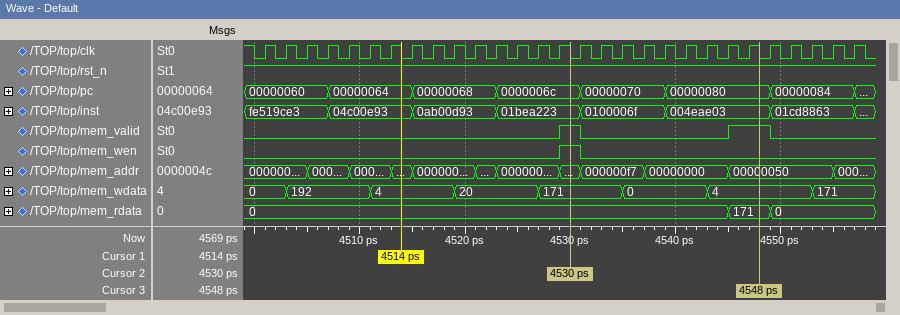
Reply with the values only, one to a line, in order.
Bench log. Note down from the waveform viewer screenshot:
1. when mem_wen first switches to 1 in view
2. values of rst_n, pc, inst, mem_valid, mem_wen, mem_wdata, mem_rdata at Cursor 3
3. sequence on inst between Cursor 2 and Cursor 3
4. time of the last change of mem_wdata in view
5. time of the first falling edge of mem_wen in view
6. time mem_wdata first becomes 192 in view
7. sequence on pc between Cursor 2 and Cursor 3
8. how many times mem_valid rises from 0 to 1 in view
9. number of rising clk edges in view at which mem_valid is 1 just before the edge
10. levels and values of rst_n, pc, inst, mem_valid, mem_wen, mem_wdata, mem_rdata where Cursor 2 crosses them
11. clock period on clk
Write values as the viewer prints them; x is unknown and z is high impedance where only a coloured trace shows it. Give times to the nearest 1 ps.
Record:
4529 ps
rst_n=1, pc=00000080, inst=004eae03, mem_valid=1, mem_wen=0, mem_wdata=4, mem_rdata=171
01bea223, 0100006f, 004eae03
4553 ps
4531 ps
4503 ps
0000006c, 00000070, 00000080
2
3
rst_n=1, pc=0000006c, inst=01bea223, mem_valid=1, mem_wen=1, mem_wdata=171, mem_rdata=0
2 ps
